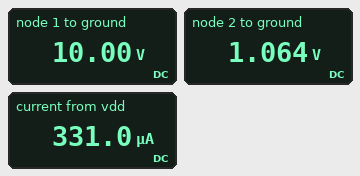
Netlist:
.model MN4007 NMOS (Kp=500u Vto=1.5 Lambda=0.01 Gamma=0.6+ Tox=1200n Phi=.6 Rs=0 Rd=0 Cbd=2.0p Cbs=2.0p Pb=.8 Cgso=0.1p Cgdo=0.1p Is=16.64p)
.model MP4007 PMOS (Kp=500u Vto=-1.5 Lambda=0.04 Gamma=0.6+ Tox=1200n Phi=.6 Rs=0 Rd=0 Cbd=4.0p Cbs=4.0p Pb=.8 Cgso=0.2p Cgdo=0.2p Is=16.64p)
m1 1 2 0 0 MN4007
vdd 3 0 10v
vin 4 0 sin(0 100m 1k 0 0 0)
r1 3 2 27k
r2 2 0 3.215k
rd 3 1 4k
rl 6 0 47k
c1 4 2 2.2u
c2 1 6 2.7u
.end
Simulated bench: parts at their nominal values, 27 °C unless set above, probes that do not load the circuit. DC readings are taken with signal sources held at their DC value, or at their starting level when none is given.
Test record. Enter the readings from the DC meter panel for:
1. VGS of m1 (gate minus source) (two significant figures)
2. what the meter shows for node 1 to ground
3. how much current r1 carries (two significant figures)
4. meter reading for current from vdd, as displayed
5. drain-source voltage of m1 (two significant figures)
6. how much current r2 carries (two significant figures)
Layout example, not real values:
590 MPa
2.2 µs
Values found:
1.1 V
10.00 V
330 µA
331.0 µA
10 V
330 µA
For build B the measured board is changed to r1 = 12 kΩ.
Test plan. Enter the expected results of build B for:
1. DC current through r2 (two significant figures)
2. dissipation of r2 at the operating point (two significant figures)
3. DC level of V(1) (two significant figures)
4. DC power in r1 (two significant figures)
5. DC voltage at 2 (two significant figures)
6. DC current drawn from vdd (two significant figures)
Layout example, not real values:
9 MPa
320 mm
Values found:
660 µA
1.4 mW
9.6 V
5.2 mW
2.1 V
760 µA
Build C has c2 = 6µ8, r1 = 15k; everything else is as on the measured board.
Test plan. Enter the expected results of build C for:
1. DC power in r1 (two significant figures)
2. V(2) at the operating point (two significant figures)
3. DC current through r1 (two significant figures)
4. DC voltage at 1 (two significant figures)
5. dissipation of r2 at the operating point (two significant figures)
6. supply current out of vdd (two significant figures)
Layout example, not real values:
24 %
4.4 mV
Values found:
4.5 mW
1.8 V
550 µA
9.9 V
970 µW
570 µA
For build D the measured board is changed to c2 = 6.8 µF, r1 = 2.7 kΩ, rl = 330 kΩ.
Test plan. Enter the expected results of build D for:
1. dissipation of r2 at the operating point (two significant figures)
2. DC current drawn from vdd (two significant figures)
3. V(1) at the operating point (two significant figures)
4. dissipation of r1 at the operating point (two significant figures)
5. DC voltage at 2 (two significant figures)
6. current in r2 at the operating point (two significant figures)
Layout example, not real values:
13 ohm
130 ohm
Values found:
9.2 mW
3.9 mA
1.3 V
7.7 mW
5.4 V
1.7 mA
